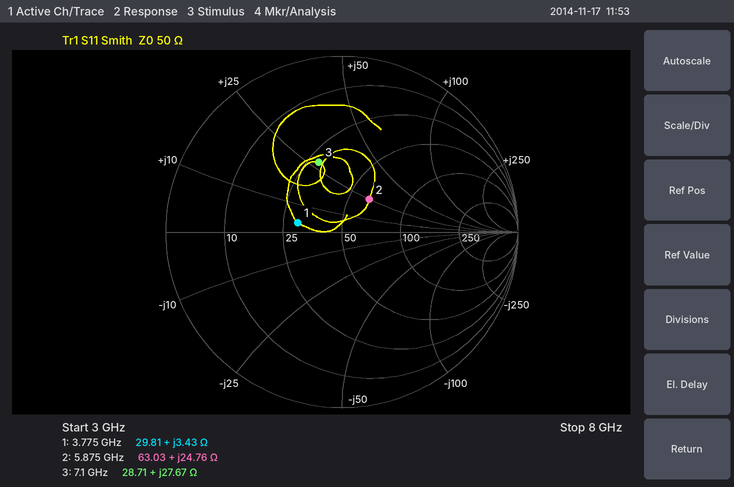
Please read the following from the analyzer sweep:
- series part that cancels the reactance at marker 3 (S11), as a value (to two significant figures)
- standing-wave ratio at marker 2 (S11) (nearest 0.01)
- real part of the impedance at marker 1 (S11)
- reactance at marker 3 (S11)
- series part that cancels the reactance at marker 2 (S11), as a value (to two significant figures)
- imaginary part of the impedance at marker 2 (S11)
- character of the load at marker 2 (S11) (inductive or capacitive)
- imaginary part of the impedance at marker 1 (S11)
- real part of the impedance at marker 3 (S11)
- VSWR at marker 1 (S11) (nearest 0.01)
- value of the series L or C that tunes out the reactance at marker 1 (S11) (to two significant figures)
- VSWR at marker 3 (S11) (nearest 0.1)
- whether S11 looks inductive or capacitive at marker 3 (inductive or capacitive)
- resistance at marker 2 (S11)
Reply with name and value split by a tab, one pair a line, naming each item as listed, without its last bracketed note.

series part that cancels the reactance at marker 3 (S11), as a value	810 fF
standing-wave ratio at marker 2 (S11)	1.64
real part of the impedance at marker 1	29.81 Ω
reactance at marker 3	+27.67 Ω
series part that cancels the reactance at marker 2 (S11), as a value	1.1 pF
imaginary part of the impedance at marker 2	+24.76 Ω
character of the load at marker 2 (S11)	inductive
imaginary part of the impedance at marker 1	+3.43 Ω
real part of the impedance at marker 3	28.71 Ω
VSWR at marker 1 (S11)	1.69
value of the series L or C that tunes out the reactance at marker 1 (S11)	12 pF
VSWR at marker 3 (S11)	2.4
whether S11 looks inductive or capacitive at marker 3	inductive
resistance at marker 2	63.03 Ω
